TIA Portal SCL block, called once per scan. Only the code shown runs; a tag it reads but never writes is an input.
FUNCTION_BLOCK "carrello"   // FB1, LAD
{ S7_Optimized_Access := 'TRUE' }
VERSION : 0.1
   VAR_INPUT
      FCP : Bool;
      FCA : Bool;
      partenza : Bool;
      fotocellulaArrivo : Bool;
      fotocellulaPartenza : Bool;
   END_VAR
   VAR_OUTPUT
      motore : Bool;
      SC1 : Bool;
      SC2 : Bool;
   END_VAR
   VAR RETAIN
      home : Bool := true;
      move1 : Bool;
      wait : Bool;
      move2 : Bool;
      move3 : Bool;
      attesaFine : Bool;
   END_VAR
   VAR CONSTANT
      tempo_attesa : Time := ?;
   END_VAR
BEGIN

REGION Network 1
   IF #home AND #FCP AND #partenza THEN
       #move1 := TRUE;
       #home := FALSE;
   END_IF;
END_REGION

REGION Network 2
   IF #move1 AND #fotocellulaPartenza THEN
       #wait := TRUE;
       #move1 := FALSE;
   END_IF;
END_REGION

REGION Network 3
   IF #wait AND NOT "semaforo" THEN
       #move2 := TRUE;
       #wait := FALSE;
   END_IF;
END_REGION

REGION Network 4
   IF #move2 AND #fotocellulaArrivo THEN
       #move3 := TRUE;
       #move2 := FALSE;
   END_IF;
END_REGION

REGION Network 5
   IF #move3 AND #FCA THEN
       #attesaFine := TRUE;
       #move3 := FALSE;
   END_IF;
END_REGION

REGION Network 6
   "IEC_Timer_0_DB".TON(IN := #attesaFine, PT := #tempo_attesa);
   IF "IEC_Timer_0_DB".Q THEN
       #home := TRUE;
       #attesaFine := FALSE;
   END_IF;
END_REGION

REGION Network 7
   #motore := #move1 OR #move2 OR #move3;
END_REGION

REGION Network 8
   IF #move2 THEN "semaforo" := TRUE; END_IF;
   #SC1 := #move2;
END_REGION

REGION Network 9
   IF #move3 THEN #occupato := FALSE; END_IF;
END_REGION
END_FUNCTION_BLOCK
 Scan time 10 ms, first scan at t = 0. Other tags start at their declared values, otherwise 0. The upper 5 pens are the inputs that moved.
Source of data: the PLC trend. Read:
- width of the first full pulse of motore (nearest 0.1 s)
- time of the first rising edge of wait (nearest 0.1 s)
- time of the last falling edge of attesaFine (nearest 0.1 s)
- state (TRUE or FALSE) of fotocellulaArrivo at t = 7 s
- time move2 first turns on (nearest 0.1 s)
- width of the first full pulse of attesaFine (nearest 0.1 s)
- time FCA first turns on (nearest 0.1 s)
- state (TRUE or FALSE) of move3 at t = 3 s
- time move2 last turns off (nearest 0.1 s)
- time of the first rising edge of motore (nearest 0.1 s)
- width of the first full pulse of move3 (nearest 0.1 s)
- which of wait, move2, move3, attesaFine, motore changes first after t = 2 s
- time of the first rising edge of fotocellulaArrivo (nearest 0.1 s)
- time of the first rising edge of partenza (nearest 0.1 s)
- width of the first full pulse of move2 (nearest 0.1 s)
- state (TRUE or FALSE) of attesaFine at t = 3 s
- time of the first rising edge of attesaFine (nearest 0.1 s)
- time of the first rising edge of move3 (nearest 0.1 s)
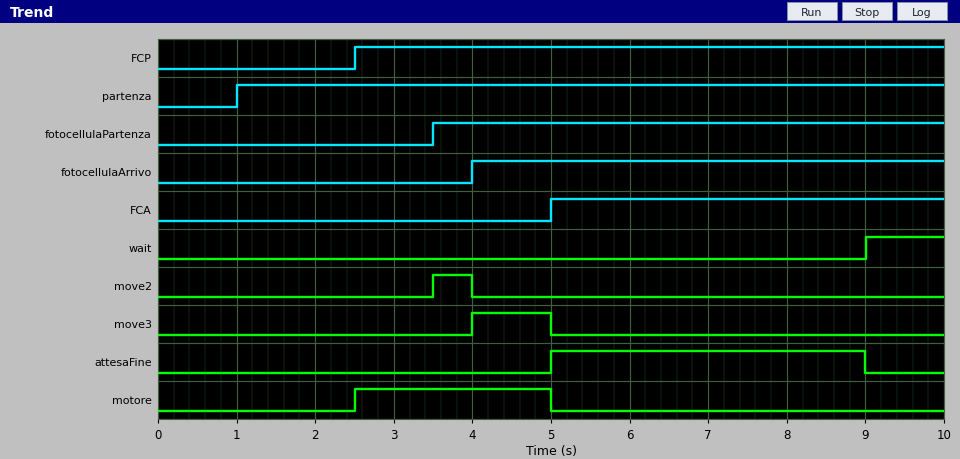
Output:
2.5 s
9.0 s
9.0 s
TRUE
3.5 s
4.0 s
5.0 s
FALSE
4.0 s
2.5 s
1.0 s
motore
4.0 s
1.0 s
0.5 s
FALSE
5.0 s
4.0 s
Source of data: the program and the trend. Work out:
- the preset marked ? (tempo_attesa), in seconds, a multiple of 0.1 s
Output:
4.0 s
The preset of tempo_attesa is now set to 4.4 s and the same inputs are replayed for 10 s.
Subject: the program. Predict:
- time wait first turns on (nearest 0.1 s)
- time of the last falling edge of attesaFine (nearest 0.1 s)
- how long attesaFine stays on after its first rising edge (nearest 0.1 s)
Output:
9.4 s
9.4 s
4.4 s
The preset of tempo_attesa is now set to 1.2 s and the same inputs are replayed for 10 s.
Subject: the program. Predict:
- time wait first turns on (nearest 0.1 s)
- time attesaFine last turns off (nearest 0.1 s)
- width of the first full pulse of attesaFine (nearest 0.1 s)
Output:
6.2 s
6.2 s
1.2 s
